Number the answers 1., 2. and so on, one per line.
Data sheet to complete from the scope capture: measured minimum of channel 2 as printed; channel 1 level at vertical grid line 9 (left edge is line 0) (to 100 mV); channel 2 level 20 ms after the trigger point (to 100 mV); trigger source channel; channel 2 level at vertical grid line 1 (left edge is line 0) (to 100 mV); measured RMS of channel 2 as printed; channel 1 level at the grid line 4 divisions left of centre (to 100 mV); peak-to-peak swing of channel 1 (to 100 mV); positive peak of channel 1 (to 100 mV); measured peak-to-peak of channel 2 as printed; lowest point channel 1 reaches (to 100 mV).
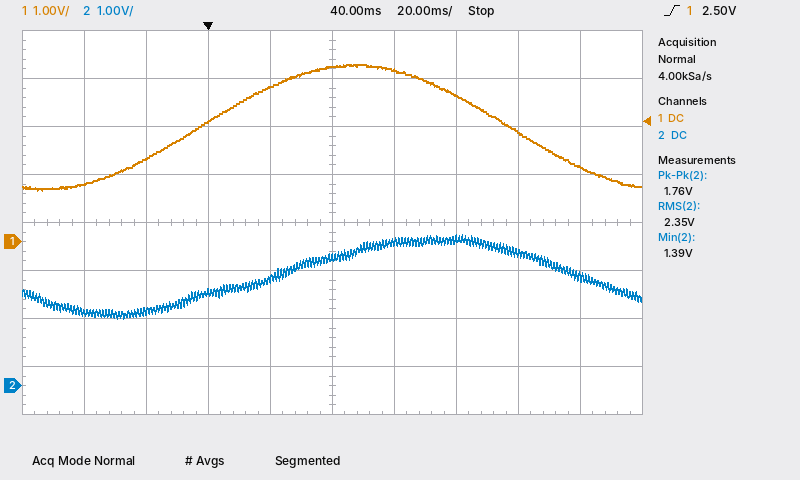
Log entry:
1. 1.39 V
2. 1.6 V
3. 2.2 V
4. channel 1
5. 1.5 V
6. 2.35 V
7. 1.2 V
8. 2.6 V
9. 3.7 V
10. 1.76 V
11. 1.1 V
